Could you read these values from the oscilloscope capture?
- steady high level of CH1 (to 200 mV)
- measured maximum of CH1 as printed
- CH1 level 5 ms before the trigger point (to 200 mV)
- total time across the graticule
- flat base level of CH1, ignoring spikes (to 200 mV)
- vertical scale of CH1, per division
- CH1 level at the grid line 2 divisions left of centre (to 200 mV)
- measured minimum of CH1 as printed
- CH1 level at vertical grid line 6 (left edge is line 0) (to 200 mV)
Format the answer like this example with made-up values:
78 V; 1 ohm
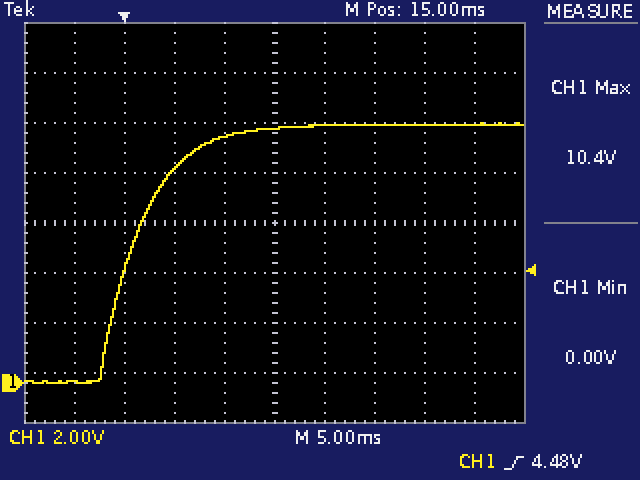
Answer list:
10.4 V; 10.4 V; 0.0 V; 50 ms; 0.0 V; 2 V; 8.6 V; 0.00 V; 10.4 V
